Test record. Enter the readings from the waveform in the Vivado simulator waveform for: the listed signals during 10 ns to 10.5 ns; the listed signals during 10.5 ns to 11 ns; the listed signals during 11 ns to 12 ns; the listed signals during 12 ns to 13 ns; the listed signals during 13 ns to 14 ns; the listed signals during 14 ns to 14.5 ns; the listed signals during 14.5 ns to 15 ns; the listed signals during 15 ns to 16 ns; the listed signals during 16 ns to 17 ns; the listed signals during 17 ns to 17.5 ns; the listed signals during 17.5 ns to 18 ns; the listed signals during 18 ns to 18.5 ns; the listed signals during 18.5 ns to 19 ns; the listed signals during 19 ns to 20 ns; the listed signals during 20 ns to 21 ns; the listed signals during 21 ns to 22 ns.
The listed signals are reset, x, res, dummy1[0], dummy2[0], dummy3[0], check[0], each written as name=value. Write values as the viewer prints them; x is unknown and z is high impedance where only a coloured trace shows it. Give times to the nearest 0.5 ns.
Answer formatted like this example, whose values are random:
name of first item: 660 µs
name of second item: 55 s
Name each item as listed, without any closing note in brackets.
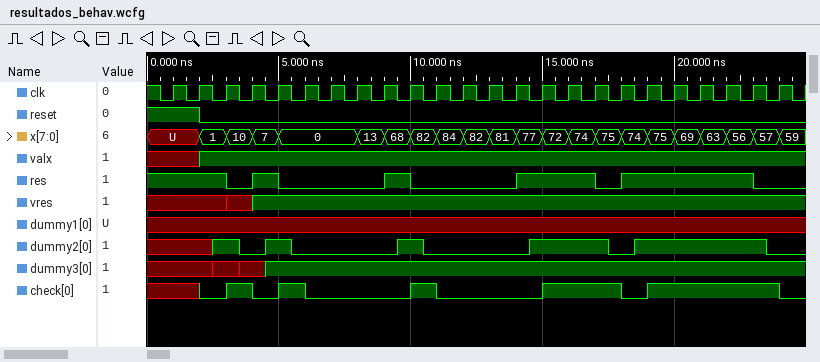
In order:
the listed signals during 10 ns to 10.5 ns: reset=0, x=82, res=0, dummy1[0]=x, dummy2[0]=1, dummy3[0]=1, check[0]=1
the listed signals during 10.5 ns to 11 ns: reset=0, x=82, res=0, dummy1[0]=x, dummy2[0]=0, dummy3[0]=1, check[0]=1
the listed signals during 11 ns to 12 ns: reset=0, x=84, res=0, dummy1[0]=x, dummy2[0]=0, dummy3[0]=1, check[0]=0
the listed signals during 12 ns to 13 ns: reset=0, x=82, res=0, dummy1[0]=x, dummy2[0]=0, dummy3[0]=1, check[0]=0
the listed signals during 13 ns to 14 ns: reset=0, x=81, res=0, dummy1[0]=x, dummy2[0]=0, dummy3[0]=1, check[0]=0
the listed signals during 14 ns to 14.5 ns: reset=0, x=77, res=1, dummy1[0]=x, dummy2[0]=0, dummy3[0]=1, check[0]=0
the listed signals during 14.5 ns to 15 ns: reset=0, x=77, res=1, dummy1[0]=x, dummy2[0]=1, dummy3[0]=1, check[0]=0
the listed signals during 15 ns to 16 ns: reset=0, x=72, res=1, dummy1[0]=x, dummy2[0]=1, dummy3[0]=1, check[0]=1
the listed signals during 16 ns to 17 ns: reset=0, x=74, res=1, dummy1[0]=x, dummy2[0]=1, dummy3[0]=1, check[0]=1
the listed signals during 17 ns to 17.5 ns: reset=0, x=75, res=0, dummy1[0]=x, dummy2[0]=1, dummy3[0]=1, check[0]=1
the listed signals during 17.5 ns to 18 ns: reset=0, x=75, res=0, dummy1[0]=x, dummy2[0]=0, dummy3[0]=1, check[0]=1
the listed signals during 18 ns to 18.5 ns: reset=0, x=74, res=1, dummy1[0]=x, dummy2[0]=0, dummy3[0]=1, check[0]=0
the listed signals during 18.5 ns to 19 ns: reset=0, x=74, res=1, dummy1[0]=x, dummy2[0]=1, dummy3[0]=1, check[0]=0
the listed signals during 19 ns to 20 ns: reset=0, x=75, res=1, dummy1[0]=x, dummy2[0]=1, dummy3[0]=1, check[0]=1
the listed signals during 20 ns to 21 ns: reset=0, x=69, res=1, dummy1[0]=x, dummy2[0]=1, dummy3[0]=1, check[0]=1
the listed signals during 21 ns to 22 ns: reset=0, x=63, res=1, dummy1[0]=x, dummy2[0]=1, dummy3[0]=1, check[0]=1
